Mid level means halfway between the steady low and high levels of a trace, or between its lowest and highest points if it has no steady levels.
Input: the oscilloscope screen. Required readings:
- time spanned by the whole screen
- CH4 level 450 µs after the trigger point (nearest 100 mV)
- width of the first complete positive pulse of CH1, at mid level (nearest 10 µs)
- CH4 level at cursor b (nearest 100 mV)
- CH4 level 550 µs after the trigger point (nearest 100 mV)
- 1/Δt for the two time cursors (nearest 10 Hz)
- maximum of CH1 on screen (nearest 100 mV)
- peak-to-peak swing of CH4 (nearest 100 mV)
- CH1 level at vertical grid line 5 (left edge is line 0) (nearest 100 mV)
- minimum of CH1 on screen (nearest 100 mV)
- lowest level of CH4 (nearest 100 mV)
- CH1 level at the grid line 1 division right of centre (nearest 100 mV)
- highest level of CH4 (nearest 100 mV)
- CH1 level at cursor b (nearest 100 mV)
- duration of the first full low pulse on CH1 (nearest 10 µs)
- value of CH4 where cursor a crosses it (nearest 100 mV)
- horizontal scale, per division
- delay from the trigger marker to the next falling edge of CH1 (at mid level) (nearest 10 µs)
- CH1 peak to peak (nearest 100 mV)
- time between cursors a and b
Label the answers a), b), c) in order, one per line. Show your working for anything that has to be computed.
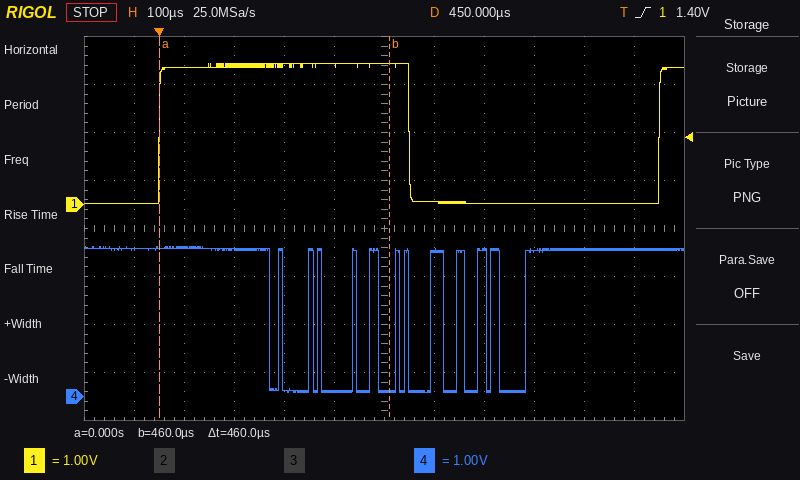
a) 1.2 ms
b) 100 mV
c) 500 µs
d) 100 mV
e) 3.0 V
f) 1 / 460 µs ≈ 2.17 kHz
g) 2.9 V
h) 3.1 V − (100 mV) = 3.0 V
i) 2.9 V
j) 0.0 V
k) 100 mV
l) 100 mV
m) 3.1 V
n) 2.9 V
o) 500 µs
p) 3.1 V
q) 100 µs
r) 500 µs
s) 2.9 V − (0.0 V) = 2.9 V
t) 460 µs
